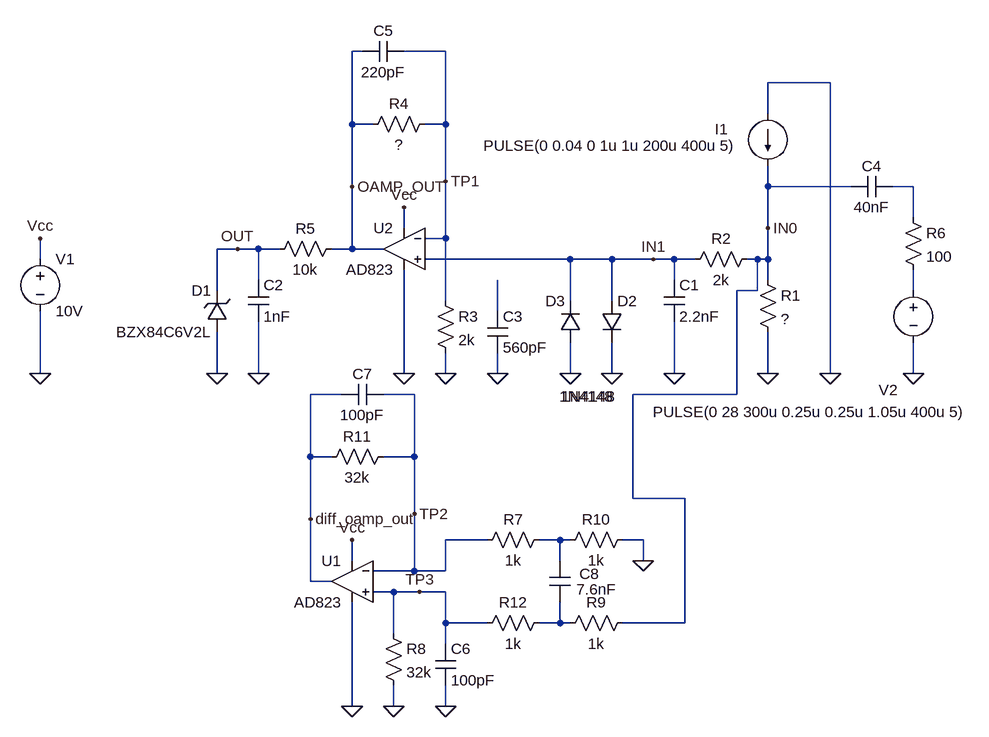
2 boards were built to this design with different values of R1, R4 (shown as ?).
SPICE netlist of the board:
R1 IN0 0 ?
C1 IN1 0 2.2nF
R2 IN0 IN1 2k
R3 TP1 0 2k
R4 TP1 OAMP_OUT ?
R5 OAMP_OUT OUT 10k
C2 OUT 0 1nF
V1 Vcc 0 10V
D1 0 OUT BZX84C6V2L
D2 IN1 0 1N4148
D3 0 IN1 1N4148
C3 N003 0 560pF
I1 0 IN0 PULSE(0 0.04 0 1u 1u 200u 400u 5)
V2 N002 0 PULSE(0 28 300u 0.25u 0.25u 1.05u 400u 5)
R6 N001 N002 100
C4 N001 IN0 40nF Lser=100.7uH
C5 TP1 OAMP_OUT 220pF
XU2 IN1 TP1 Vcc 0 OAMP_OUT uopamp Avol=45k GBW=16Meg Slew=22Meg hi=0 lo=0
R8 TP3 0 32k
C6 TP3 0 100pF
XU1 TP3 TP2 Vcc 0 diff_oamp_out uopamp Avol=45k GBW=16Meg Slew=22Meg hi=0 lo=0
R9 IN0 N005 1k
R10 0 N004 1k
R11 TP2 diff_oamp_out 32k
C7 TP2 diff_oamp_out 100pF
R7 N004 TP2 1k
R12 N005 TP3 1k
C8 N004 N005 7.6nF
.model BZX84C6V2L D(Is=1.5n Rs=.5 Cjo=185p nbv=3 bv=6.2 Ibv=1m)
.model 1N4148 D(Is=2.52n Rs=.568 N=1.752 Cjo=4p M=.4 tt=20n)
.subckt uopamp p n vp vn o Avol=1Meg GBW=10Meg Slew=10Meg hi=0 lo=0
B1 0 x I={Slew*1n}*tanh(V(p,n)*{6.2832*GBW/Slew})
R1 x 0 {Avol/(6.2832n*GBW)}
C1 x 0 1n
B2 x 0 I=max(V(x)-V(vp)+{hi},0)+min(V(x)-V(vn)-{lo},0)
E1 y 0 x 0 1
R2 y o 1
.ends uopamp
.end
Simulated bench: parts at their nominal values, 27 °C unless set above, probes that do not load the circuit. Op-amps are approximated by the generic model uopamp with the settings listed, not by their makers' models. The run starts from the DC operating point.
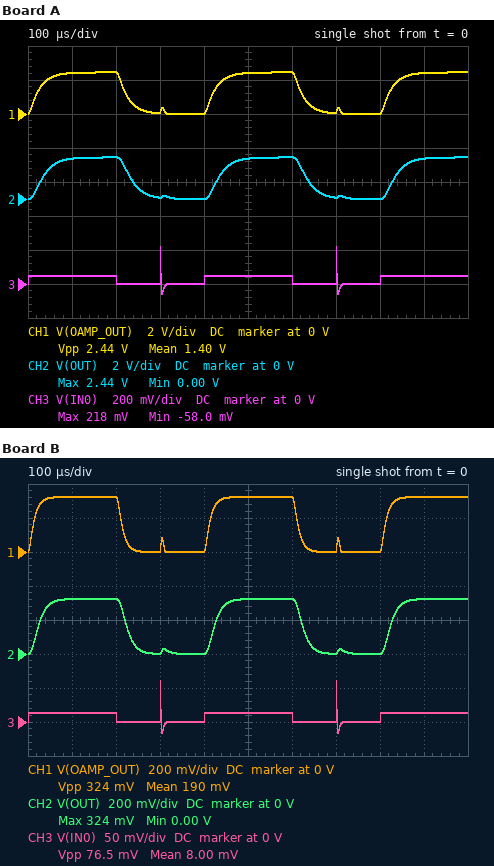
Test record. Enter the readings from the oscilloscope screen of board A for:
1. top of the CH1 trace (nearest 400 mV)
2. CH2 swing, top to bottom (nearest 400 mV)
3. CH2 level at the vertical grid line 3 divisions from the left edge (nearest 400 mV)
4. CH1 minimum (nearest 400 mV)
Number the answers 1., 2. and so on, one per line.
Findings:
1. 2.4 V
2. 2.4 V
3. 0 V
4. 0 V
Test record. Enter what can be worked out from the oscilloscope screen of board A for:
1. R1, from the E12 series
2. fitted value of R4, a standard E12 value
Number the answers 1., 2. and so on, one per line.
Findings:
1. 1.2 Ω
2. 100 kΩ
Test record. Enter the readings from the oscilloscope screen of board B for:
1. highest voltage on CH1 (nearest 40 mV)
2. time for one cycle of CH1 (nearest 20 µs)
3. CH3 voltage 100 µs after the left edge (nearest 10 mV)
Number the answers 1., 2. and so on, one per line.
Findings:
1. 320 mV
2. 400 µs
3. 10 mV
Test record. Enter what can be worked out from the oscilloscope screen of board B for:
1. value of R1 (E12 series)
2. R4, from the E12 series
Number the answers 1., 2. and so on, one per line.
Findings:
1. 0.33 Ω
2. 47 kΩ
